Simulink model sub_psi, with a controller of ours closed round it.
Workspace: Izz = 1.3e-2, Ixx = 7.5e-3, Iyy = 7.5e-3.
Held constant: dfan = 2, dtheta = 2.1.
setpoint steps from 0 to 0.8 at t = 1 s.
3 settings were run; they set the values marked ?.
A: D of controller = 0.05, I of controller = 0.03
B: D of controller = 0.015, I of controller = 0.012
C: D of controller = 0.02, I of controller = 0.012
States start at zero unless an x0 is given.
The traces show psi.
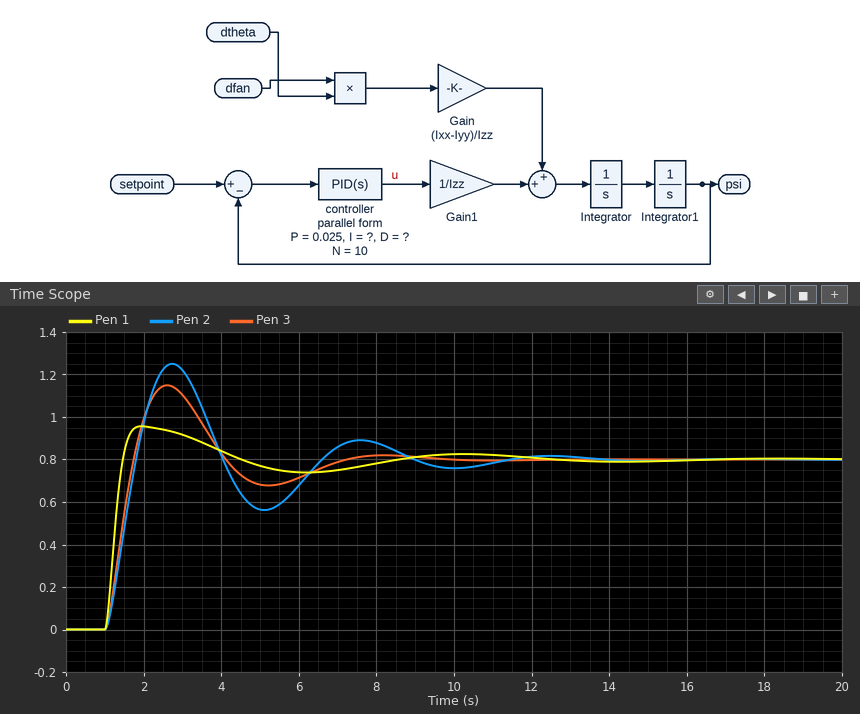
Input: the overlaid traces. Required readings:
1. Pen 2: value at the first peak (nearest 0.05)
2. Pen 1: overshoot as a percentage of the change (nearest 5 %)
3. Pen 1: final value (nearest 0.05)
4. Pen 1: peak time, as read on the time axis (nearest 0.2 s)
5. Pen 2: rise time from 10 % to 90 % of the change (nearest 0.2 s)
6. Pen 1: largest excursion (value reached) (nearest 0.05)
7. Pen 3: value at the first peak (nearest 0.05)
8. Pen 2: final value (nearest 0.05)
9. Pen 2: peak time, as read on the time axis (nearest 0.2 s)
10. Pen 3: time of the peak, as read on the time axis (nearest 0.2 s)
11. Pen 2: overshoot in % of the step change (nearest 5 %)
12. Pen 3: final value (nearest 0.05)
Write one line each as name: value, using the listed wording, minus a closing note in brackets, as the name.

Pen 2: value at the first peak: 1.25
Pen 1: overshoot as a percentage of the change: 20 %
Pen 1: final value: 0.80
Pen 1: peak time, as read on the time axis: 2.0 s
Pen 2: rise time from 10 % to 90 % of the change: 0.6 s
Pen 1: largest excursion (value reached): 0.95
Pen 3: value at the first peak: 1.15
Pen 2: final value: 0.80
Pen 2: peak time, as read on the time axis: 2.8 s
Pen 3: time of the peak, as read on the time axis: 2.6 s
Pen 2: overshoot in % of the step change: 55 %
Pen 3: final value: 0.80
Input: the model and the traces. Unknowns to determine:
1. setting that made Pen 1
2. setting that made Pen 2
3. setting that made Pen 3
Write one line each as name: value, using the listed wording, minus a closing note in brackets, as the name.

setting that made Pen 1: A
setting that made Pen 2: B
setting that made Pen 3: C
